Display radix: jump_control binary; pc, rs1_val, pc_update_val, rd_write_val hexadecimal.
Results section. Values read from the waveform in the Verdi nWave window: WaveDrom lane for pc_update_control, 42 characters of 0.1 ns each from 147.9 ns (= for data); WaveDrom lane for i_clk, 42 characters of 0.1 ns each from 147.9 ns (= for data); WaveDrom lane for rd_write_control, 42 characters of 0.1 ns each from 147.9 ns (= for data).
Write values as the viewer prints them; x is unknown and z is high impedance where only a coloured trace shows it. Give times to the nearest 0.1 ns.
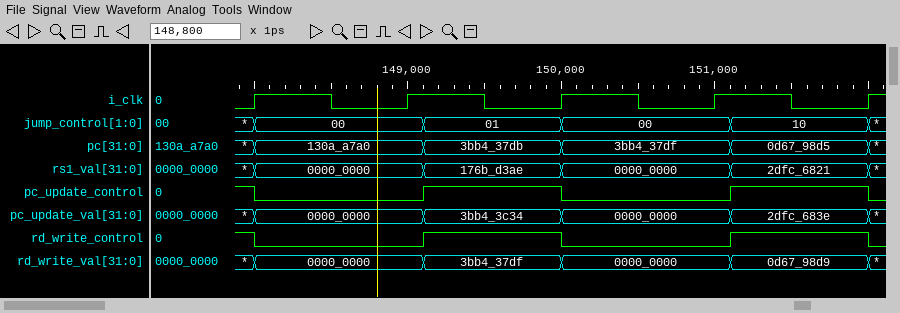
{name: 'pc_update_control', wave: '10..........1........0..........1........0'}
{name: 'i_clk', wave: '01....0....1....0....1....0....1....0....1'}
{name: 'rd_write_control', wave: '10..........1........0..........1........0'}
